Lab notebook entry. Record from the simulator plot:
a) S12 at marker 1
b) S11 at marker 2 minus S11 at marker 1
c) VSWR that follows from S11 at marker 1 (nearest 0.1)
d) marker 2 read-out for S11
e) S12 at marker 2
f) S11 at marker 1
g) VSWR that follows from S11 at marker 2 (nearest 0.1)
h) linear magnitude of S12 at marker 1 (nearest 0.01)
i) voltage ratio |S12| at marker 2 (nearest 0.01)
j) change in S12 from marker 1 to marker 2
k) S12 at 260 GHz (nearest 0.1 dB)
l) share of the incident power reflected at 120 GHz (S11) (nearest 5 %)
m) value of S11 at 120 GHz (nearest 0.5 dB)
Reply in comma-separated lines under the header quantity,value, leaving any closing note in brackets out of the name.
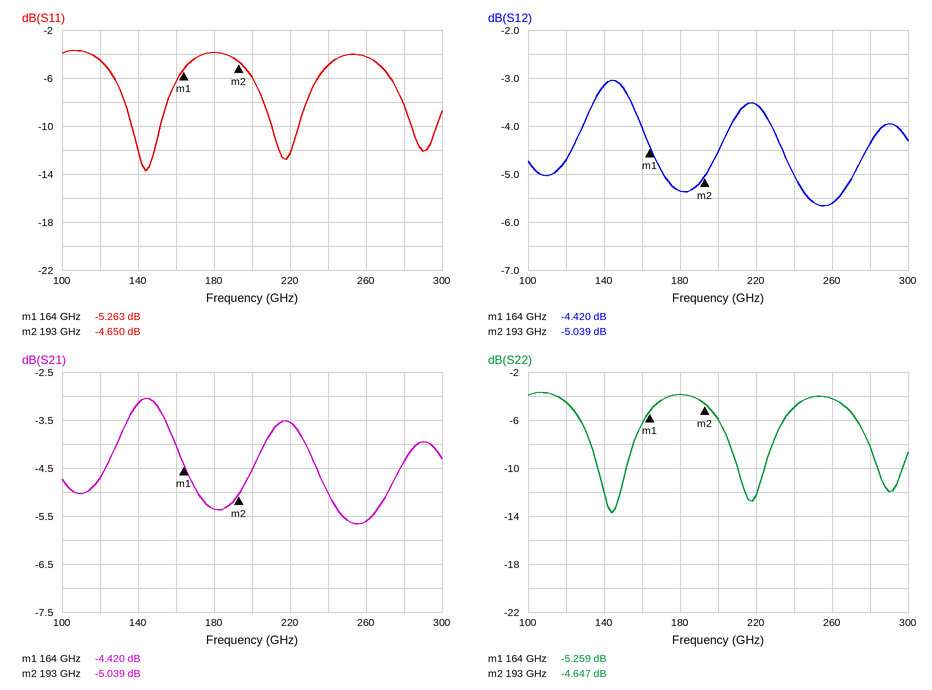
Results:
quantity,value
S12 at marker 1,-4.420 dB
S11 at marker 2 minus S11 at marker 1,0.613 dB
VSWR that follows from S11 at marker 1,3.4
marker 2 read-out for S11,-4.650 dB
S12 at marker 2,-5.039 dB
S11 at marker 1,-5.263 dB
VSWR that follows from S11 at marker 2,3.8
linear magnitude of S12 at marker 1,0.60
voltage ratio |S12| at marker 2,0.56
change in S12 from marker 1 to marker 2,-0.619 dB
S12 at 260 GHz,-5.6 dB
share of the incident power reflected at 120 GHz (S11),35 %
value of S11 at 120 GHz,-4.5 dB
